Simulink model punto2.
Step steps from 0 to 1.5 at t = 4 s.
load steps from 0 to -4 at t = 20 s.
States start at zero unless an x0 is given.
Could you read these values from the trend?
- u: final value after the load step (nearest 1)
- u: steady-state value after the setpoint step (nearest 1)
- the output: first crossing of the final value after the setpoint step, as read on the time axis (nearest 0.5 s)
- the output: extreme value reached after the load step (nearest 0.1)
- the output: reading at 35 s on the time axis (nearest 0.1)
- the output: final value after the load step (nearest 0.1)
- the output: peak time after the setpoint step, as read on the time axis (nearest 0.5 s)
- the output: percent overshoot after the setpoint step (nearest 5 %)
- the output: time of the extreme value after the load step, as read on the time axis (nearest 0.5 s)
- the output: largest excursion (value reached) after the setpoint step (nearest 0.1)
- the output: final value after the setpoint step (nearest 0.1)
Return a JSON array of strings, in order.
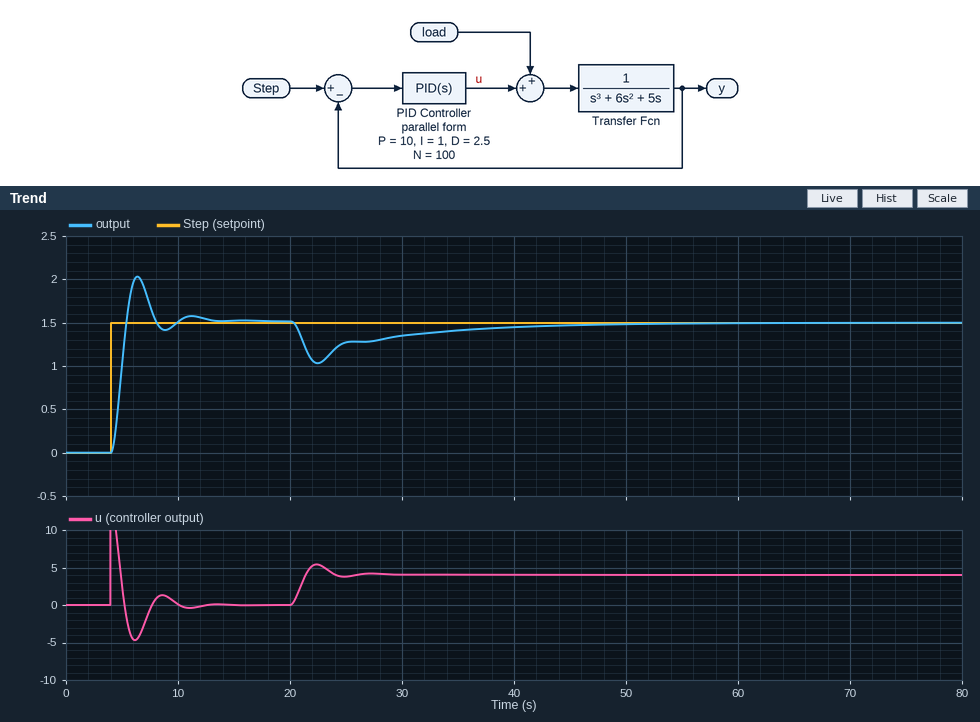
["4", "0", "5.5 s", "1.0", "1.4", "1.5", "6.5 s", "35 %", "22.5 s", "2.0", "1.5"]
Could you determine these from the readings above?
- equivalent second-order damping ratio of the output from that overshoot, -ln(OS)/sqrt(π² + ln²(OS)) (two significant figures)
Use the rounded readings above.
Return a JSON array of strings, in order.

["0.32"]
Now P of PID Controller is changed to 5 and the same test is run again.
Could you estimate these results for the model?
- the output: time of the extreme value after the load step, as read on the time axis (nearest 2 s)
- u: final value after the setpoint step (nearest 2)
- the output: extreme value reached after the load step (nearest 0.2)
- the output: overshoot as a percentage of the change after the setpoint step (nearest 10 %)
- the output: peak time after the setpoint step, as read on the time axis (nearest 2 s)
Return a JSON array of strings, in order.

["24 s", "0", "0.8", "30 %", "8 s"]
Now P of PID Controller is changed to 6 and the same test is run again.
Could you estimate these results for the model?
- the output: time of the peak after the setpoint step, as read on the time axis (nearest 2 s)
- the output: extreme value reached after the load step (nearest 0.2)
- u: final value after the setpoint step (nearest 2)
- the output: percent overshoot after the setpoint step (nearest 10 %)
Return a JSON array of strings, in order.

["8 s", "0.8", "0", "30 %"]
